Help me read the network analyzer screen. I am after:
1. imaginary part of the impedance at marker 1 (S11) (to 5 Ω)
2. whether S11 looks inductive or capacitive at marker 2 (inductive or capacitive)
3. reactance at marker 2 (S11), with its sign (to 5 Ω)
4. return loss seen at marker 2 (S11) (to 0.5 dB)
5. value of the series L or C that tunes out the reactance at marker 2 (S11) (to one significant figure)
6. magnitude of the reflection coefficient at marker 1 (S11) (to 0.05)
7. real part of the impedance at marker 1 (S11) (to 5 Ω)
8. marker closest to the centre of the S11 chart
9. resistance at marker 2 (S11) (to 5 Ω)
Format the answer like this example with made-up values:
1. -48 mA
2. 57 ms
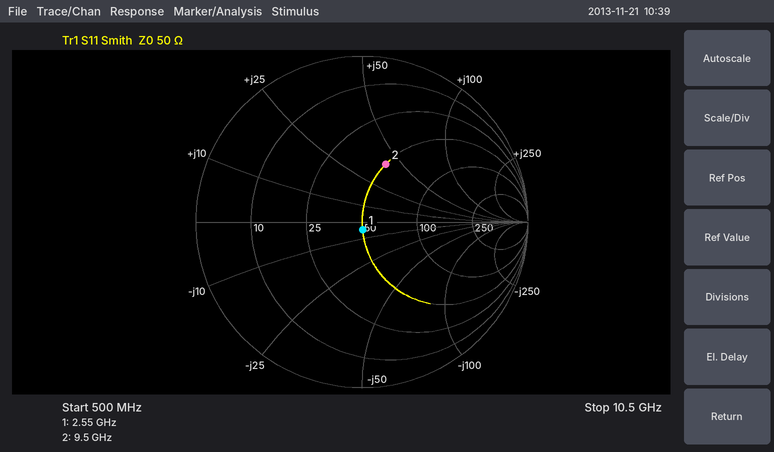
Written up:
1. -5 Ω
2. inductive
3. +40 Ω
4. 8.5 dB
5. 400 fF
6. 0.05
7. 50 Ω
8. marker 1
9. 50 Ω
